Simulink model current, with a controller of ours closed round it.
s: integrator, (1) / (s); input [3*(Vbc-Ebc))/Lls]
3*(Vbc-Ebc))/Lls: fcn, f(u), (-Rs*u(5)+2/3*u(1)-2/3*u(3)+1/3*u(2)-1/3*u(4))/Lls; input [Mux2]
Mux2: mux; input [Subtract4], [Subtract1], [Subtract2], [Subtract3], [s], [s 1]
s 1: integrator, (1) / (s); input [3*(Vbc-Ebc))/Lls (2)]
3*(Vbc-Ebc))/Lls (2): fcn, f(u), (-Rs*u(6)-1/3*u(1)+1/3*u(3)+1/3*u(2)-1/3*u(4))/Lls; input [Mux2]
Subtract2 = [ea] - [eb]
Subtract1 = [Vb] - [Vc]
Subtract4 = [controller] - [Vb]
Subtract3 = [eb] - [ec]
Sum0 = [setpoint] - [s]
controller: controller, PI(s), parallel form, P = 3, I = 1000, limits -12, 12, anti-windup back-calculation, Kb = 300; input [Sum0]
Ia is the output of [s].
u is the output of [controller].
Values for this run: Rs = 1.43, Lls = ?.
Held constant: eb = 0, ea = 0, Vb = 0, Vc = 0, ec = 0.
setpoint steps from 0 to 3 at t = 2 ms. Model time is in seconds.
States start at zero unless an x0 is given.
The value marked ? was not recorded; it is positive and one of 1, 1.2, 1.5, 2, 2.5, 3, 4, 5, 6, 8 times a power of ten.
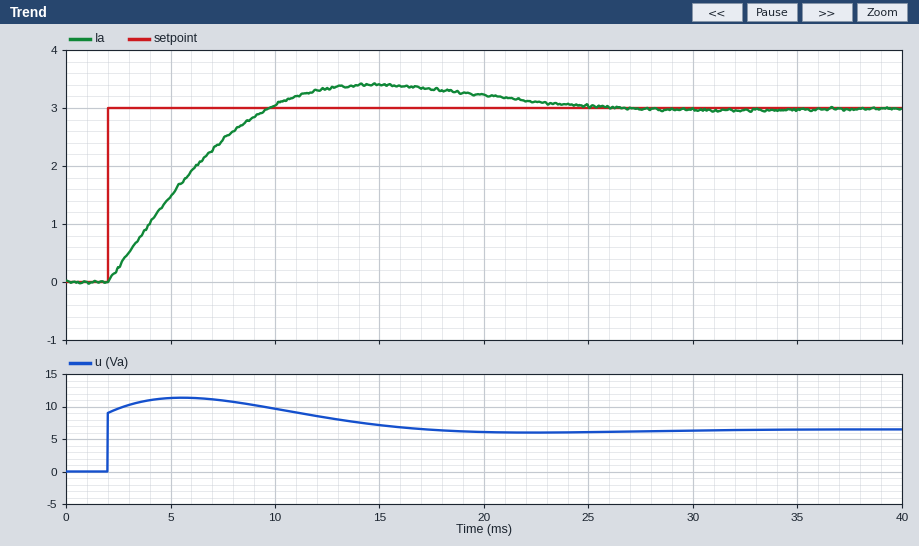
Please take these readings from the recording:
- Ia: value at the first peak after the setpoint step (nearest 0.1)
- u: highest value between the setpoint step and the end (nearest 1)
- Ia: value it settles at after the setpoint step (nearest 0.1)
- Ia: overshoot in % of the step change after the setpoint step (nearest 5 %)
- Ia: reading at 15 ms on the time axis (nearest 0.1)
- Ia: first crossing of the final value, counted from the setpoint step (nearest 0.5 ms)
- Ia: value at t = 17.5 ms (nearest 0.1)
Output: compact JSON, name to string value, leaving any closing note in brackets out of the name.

{"Ia: value at the first peak after the setpoint step": "3.4", "u: highest value between the setpoint step and the end": "11", "Ia: value it settles at after the setpoint step": "3.0", "Ia: overshoot in % of the step change after the setpoint step": "15 %", "Ia: reading at 15 ms on the time axis": "3.4", "Ia: first crossing of the final value, counted from the setpoint step": "7.5 ms", "Ia: value at t = 17.5 ms": "3.3"}
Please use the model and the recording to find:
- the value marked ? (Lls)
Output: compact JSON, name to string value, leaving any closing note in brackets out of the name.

{"the value marked ?": "0.012"}
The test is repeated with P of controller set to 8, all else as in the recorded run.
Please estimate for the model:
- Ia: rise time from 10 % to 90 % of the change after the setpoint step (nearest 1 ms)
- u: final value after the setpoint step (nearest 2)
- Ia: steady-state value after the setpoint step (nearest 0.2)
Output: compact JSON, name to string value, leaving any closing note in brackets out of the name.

{"Ia: rise time from 10 % to 90 % of the change after the setpoint step": "7 ms", "u: final value after the setpoint step": "6", "Ia: steady-state value after the setpoint step": "3.0"}
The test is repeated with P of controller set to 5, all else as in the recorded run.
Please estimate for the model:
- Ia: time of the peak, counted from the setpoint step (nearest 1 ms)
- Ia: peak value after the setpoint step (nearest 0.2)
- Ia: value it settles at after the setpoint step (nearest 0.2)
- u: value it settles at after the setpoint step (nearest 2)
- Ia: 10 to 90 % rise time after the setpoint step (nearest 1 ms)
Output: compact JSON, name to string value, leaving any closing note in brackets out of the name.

{"Ia: time of the peak, counted from the setpoint step": "13 ms", "Ia: peak value after the setpoint step": "3.2", "Ia: value it settles at after the setpoint step": "3.0", "u: value it settles at after the setpoint step": "6", "Ia: 10 to 90 % rise time after the setpoint step": "6 ms"}
